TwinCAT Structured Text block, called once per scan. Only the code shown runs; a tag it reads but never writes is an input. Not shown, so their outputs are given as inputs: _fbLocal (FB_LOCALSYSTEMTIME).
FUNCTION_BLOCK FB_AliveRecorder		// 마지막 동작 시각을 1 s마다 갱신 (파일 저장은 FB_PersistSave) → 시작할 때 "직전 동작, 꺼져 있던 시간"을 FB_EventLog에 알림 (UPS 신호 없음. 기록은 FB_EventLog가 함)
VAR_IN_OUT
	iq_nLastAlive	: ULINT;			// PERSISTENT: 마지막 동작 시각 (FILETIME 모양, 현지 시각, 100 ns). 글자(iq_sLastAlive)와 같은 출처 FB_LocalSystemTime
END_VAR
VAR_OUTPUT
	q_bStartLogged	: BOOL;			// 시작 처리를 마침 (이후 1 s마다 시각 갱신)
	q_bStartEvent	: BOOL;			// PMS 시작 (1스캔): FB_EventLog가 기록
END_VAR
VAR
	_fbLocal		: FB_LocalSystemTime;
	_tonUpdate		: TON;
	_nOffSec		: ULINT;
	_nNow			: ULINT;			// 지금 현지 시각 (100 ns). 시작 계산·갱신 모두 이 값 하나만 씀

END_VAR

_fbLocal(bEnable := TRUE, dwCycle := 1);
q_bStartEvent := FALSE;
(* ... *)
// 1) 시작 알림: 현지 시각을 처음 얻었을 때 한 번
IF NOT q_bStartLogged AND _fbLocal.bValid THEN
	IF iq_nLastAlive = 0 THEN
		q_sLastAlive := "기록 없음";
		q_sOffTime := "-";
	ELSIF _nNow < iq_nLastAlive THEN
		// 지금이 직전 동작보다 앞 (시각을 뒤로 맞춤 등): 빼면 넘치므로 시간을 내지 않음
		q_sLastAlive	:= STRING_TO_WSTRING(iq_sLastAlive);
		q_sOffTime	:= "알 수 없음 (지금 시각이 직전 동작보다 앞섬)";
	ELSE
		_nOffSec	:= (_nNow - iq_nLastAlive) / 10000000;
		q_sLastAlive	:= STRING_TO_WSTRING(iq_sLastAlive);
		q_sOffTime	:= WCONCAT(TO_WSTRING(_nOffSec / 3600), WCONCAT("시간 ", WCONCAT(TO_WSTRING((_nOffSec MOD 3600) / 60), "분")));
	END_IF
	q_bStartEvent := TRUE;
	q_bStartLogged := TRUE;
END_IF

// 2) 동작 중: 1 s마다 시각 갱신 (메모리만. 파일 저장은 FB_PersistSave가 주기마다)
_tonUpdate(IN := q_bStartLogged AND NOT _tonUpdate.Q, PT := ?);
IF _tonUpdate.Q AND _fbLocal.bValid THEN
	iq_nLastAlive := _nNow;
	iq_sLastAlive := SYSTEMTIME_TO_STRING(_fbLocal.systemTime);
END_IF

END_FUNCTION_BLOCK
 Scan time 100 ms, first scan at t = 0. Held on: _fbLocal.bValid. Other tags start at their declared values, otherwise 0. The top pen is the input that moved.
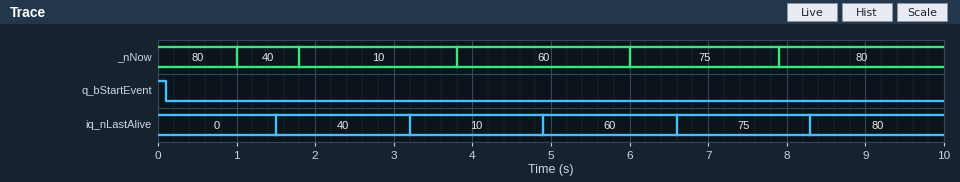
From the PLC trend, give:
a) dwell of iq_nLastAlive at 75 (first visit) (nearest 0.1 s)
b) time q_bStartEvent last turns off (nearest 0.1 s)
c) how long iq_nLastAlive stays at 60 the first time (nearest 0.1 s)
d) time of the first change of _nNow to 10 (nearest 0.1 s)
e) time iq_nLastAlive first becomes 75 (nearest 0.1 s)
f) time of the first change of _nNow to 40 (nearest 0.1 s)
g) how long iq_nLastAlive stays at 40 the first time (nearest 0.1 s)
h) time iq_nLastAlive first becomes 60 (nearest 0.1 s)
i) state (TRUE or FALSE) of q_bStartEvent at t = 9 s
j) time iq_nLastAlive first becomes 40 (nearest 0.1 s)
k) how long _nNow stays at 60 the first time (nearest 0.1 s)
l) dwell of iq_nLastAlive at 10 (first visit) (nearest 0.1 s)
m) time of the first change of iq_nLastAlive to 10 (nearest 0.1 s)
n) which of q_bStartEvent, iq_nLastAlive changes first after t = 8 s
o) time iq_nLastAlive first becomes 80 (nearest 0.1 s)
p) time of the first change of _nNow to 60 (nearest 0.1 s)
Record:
1.7 s
0.1 s
1.7 s
1.8 s
6.6 s
1.0 s
1.7 s
4.9 s
FALSE
1.5 s
2.2 s
1.7 s
3.2 s
iq_nLastAlive
8.3 s
3.8 s
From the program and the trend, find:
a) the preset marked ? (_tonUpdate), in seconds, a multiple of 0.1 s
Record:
1.5 s
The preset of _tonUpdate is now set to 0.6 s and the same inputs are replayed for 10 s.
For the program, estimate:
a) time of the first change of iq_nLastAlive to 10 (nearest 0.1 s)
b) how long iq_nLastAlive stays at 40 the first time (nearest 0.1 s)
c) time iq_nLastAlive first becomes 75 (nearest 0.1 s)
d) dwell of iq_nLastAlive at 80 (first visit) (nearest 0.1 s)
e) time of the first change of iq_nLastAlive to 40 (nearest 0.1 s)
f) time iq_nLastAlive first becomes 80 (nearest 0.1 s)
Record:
2.2 s
0.8 s
6.2 s
0.8 s
1.4 s
0.6 s
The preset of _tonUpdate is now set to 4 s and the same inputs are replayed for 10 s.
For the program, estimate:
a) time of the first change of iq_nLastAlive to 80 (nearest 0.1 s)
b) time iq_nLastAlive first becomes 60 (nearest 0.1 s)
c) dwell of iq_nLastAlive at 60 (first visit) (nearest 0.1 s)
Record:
8.2 s
4.0 s
4.2 s
